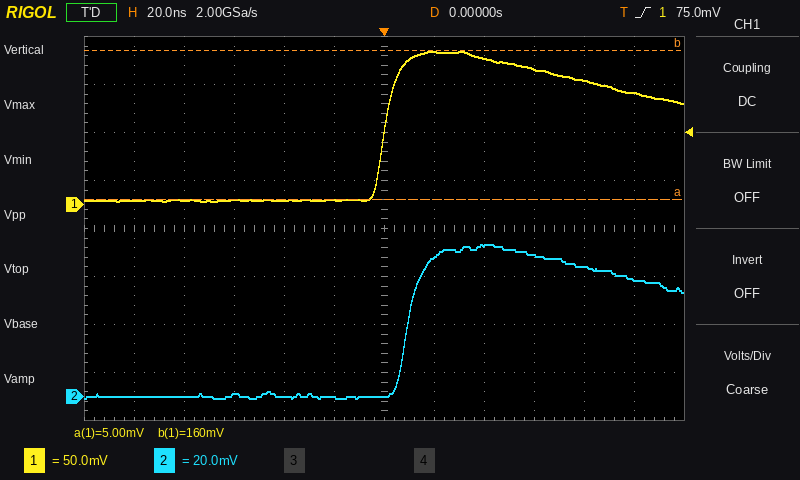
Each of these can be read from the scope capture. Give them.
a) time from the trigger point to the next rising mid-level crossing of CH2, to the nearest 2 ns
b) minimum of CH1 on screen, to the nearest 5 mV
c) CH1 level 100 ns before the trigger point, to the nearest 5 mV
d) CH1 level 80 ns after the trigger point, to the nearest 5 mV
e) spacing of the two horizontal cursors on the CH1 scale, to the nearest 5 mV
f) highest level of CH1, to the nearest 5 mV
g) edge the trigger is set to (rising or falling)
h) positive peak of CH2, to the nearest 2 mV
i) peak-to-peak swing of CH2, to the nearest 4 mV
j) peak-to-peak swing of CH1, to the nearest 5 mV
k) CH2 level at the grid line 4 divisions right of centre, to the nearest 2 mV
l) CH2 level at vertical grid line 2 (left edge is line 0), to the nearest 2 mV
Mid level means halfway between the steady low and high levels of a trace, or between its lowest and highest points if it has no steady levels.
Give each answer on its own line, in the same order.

10 ns
5 mV
5 mV
130 mV
155 mV
160 mV
rising
64 mV
64 mV
155 mV
54 mV
0 mV
